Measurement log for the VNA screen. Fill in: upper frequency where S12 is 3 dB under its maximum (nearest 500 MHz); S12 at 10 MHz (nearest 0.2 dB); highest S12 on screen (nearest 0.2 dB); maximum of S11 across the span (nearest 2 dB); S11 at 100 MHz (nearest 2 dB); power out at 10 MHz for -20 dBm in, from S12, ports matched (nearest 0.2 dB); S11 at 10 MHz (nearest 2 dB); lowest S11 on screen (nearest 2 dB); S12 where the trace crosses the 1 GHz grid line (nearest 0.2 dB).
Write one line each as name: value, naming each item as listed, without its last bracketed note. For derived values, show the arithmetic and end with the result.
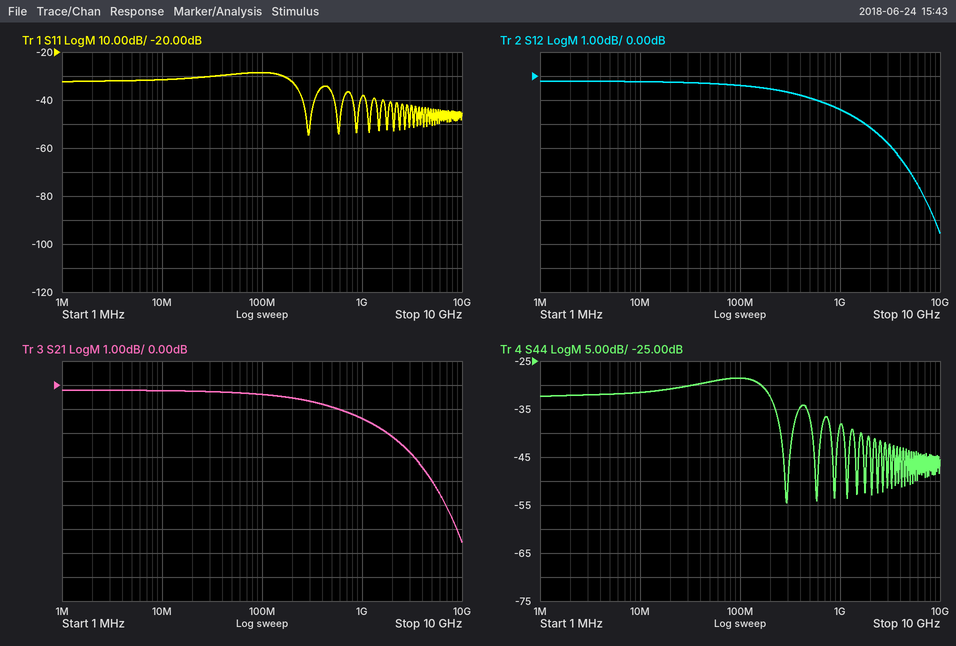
upper frequency where S12 is 3 dB under its maximum: 3.5 GHz
S12 at 10 MHz: -0.2 dB
highest S12 on screen: -0.2 dB
maximum of S11 across the span: -28 dB
S11 at 100 MHz: -28 dB
power out at 10 MHz for -20 dBm in, from S12, ports matched: -20 dBm + (-0.2 dB) = -20.2 dBm
S11 at 10 MHz: -32 dB
lowest S11 on screen: -54 dB
S12 where the trace crosses the 1 GHz grid line: -1.4 dB
